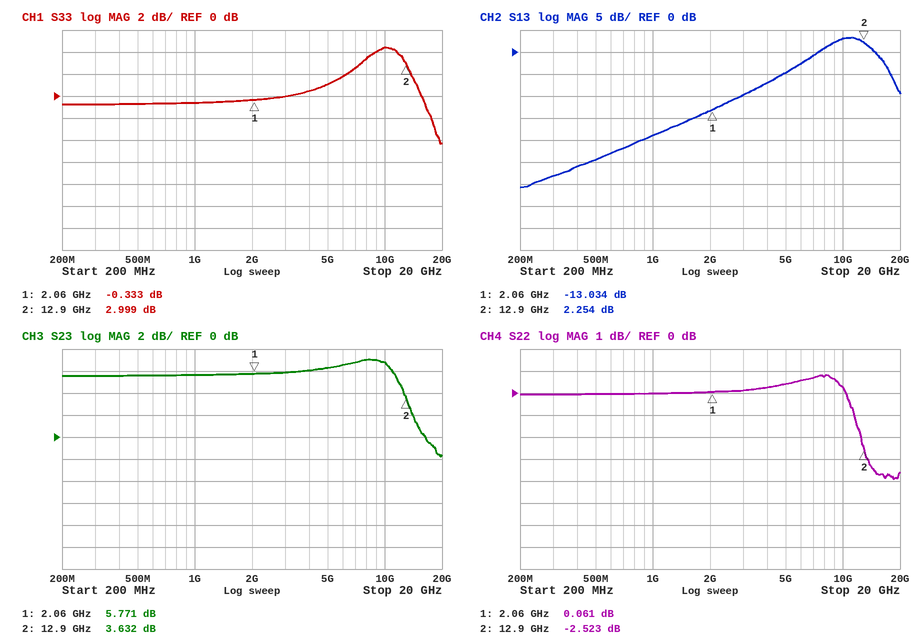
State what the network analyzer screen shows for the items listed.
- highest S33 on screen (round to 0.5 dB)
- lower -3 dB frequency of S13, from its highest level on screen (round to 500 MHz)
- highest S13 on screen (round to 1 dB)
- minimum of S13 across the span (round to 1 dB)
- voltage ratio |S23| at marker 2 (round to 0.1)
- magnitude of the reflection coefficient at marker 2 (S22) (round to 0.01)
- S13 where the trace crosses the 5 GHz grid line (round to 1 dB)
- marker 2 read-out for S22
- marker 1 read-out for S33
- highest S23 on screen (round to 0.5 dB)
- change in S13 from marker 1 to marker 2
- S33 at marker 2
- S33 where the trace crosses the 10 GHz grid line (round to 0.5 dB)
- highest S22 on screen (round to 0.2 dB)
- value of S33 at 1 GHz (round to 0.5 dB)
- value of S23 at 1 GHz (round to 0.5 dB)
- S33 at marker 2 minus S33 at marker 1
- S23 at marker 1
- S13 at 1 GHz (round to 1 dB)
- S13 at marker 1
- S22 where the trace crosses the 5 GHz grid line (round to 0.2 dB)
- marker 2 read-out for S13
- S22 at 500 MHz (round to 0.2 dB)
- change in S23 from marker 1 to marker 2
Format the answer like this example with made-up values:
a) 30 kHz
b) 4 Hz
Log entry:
a) 4.5 dB
b) 7.5 GHz
c) 3 dB
d) -31 dB
e) 1.5
f) 0.75
g) -5 dB
h) -2.523 dB
i) -0.333 dB
j) 7.0 dB
k) 15.288 dB
l) 2.999 dB
m) 4.5 dB
n) 0.8 dB
o) -0.5 dB
p) 5.5 dB
q) 3.332 dB
r) 5.771 dB
s) -19 dB
t) -13.034 dB
u) 0.4 dB
v) 2.254 dB
w) 0.0 dB
x) -2.139 dB
